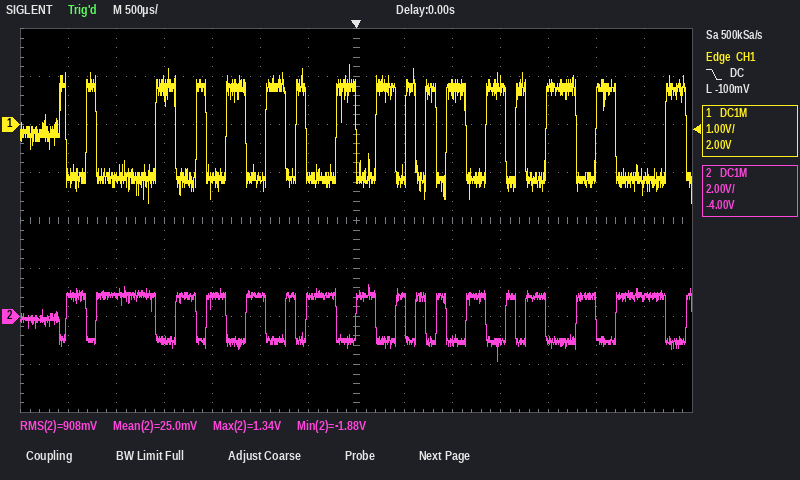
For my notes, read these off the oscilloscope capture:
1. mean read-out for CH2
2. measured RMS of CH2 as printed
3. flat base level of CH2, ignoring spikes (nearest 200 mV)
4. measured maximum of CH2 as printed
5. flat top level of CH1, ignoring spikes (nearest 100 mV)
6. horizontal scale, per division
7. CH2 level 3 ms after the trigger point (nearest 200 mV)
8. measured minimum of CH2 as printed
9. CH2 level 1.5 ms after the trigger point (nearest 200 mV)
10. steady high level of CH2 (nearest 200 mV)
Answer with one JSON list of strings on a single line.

["25.0 mV", "908 mV", "-1.0 V", "1.34 V", "800 mV", "500 µs", "800 mV", "-1.88 V", "-1.0 V", "800 mV"]
